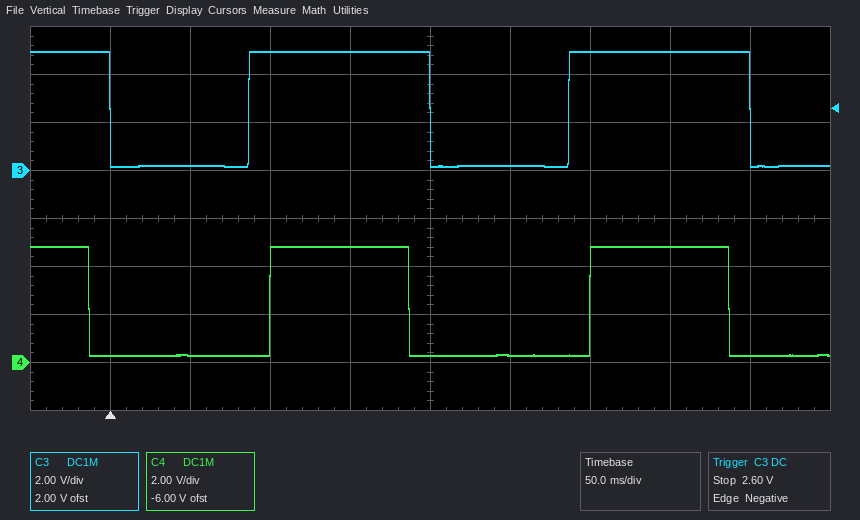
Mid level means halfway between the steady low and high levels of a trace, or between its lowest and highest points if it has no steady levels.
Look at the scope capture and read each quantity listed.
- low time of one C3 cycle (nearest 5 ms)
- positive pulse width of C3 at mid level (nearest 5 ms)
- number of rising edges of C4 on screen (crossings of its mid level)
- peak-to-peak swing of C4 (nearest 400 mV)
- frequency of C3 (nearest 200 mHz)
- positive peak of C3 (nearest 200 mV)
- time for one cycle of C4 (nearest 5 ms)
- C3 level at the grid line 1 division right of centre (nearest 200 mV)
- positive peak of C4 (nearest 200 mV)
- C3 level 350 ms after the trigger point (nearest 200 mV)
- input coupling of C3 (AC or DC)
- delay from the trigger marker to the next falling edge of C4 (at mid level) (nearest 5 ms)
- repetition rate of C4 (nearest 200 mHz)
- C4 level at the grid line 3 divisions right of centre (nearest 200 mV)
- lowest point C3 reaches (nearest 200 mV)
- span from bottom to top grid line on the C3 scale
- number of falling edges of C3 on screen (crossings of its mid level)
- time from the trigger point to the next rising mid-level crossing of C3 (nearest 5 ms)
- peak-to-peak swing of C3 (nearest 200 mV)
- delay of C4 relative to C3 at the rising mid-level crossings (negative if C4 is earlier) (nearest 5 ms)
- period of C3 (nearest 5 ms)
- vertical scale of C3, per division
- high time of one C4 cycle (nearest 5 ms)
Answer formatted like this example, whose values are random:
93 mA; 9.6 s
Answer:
85 ms; 115 ms; 2; 4.4 V; 5.0 Hz; 5.0 V; 200 ms; 200 mV; 4.8 V; 5.0 V; DC; 185 ms; 5.0 Hz; 4.8 V; 200 mV; 16 V; 3; 85 ms; 4.8 V; +15 ms; 200 ms; 2 V; 85 ms
